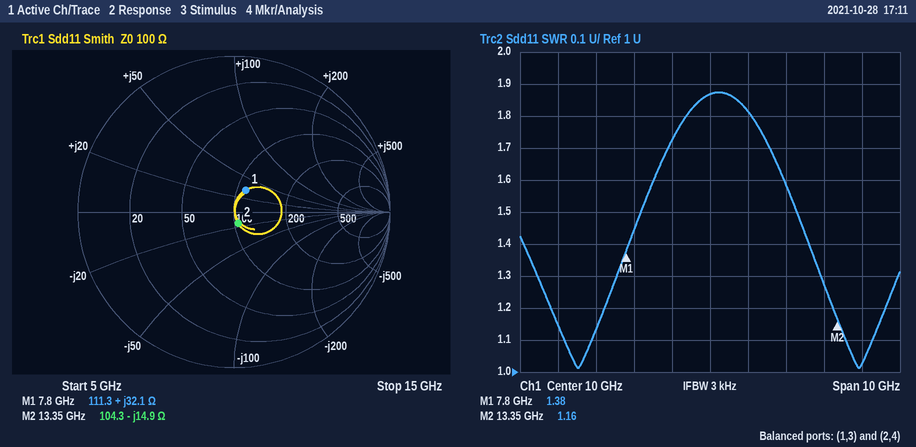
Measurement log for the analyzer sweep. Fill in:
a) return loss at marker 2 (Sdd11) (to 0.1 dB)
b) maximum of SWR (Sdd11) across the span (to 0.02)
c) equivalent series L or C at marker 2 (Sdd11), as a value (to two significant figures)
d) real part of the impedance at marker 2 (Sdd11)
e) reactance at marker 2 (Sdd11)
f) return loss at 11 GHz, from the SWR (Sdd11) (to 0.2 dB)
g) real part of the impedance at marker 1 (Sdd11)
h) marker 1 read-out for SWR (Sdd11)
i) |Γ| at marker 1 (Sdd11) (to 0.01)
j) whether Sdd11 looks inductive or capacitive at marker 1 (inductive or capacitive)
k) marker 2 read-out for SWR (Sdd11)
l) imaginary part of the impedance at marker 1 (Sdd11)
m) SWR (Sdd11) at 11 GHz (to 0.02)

22.4 dB
1.88
800 fF
104.3 Ω
-14.9 Ω
10.8 dB
111.3 Ω
1.38
0.16
inductive
1.16
+32.1 Ω
1.82
